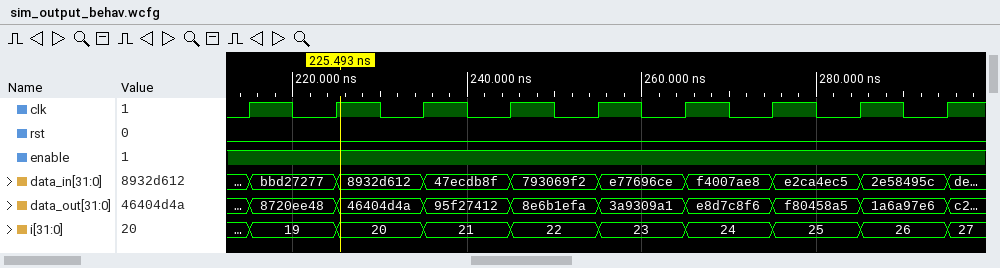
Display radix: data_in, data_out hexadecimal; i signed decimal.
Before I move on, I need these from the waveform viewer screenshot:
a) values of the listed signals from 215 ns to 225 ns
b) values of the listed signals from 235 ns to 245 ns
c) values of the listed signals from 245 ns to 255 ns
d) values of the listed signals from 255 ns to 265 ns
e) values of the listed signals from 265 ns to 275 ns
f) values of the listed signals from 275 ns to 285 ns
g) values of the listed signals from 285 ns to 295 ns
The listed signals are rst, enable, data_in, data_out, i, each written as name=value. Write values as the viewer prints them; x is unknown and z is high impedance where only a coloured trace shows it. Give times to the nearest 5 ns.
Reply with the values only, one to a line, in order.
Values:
rst=0, enable=1, data_in=bbd27277, data_out=8720ee48, i=19
rst=0, enable=1, data_in=47ecdb8f, data_out=95f27412, i=21
rst=0, enable=1, data_in=793069f2, data_out=8e6b1efa, i=22
rst=0, enable=1, data_in=e77696ce, data_out=3a9309a1, i=23
rst=0, enable=1, data_in=f4007ae8, data_out=e8d7c8f6, i=24
rst=0, enable=1, data_in=e2ca4ec5, data_out=f80458a5, i=25
rst=0, enable=1, data_in=2e58495c, data_out=1a6a97e6, i=26
